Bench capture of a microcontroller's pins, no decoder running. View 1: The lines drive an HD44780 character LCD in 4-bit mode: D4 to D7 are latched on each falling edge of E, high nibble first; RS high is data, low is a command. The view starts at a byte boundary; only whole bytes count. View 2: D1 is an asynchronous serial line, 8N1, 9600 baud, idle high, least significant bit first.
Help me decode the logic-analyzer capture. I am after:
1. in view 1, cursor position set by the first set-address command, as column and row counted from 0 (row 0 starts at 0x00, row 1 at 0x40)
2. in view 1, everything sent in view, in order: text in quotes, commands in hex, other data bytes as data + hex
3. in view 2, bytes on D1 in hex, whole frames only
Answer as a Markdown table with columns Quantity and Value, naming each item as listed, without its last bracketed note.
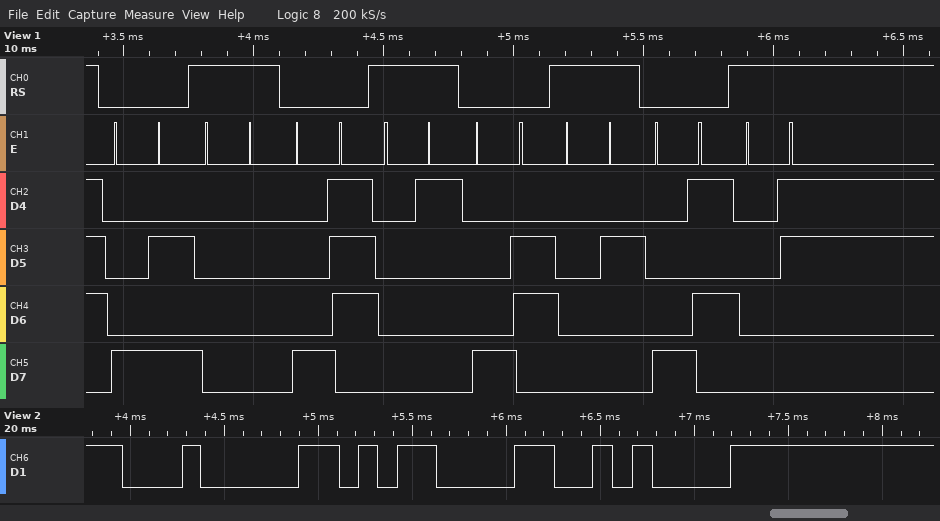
| Quantity | Value |
|---|---|
| in view 1, cursor position set by the first set-address command, as column and row counted from 0 | column 10, row 0 |
| in view 1, everything sent in view, in order: text in quotes, commands in hex, other data bytes as data + hex | 0x8A data 00 0x87 data 01 0x86 data 02 0x85 data 03 |
| in view 2, bytes on D1 in hex, whole frames only | 04 0D 0A |
